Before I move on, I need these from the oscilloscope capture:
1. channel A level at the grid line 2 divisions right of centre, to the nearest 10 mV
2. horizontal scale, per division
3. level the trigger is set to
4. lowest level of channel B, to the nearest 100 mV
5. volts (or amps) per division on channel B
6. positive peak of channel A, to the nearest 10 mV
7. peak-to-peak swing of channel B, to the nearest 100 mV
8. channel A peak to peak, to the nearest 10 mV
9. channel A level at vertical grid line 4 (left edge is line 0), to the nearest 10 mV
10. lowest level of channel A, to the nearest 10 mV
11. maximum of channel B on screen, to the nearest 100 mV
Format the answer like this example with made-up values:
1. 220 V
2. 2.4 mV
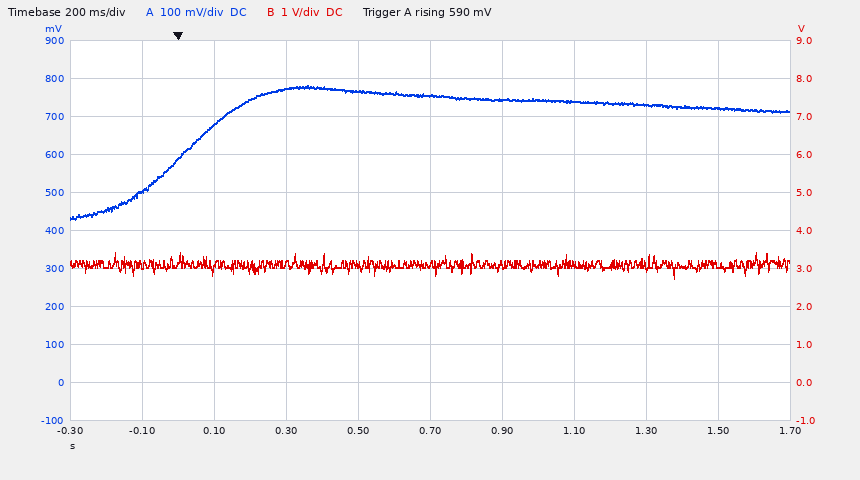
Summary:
1. 740 mV
2. 200 ms
3. 590 mV
4. 2.7 V
5. 1 V
6. 780 mV
7. 700 mV
8. 350 mV
9. 770 mV
10. 430 mV
11. 3.4 V
